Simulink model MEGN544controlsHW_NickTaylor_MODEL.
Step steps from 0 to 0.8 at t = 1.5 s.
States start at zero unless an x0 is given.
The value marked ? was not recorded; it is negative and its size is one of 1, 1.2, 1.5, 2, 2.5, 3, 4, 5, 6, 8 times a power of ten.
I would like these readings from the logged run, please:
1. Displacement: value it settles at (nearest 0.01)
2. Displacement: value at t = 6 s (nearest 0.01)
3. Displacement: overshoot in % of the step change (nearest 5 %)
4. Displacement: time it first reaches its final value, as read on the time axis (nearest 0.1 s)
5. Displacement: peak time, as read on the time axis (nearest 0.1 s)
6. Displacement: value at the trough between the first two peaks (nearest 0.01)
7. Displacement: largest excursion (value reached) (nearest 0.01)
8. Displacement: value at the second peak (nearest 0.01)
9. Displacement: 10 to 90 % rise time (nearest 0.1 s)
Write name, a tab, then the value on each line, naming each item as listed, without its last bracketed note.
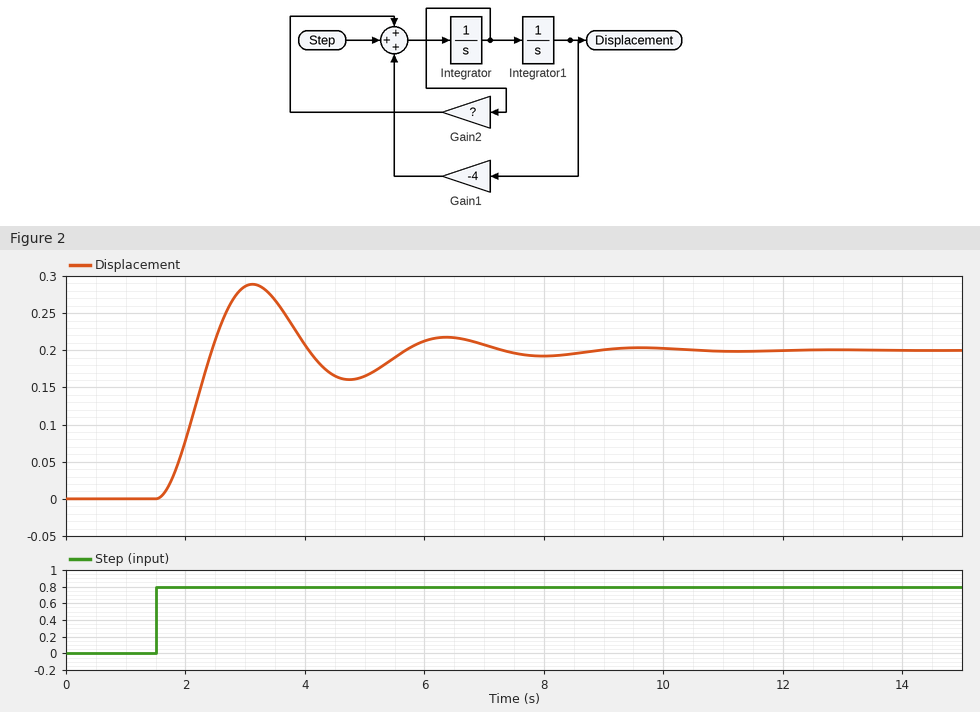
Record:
Displacement: value it settles at	0.20
Displacement: value at t = 6 s	0.21
Displacement: overshoot in % of the step change	45 %
Displacement: time it first reaches its final value, as read on the time axis	2.4 s
Displacement: peak time, as read on the time axis	3.1 s
Displacement: value at the trough between the first two peaks	0.16
Displacement: largest excursion (value reached)	0.29
Displacement: value at the second peak	0.22
Displacement: 10 to 90 % rise time	0.6 s
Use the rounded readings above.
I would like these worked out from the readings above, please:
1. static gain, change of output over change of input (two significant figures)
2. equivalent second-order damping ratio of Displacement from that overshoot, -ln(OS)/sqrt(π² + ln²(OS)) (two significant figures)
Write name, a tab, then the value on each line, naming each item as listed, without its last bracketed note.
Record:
static gain, change of output over change of input	0.25
equivalent second-order damping ratio of Displacement from that overshoot, -ln(OS)/sqrt(π² + ln²(OS))	0.25
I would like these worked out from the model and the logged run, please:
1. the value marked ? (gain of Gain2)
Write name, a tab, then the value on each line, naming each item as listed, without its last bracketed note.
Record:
the value marked ?	-1
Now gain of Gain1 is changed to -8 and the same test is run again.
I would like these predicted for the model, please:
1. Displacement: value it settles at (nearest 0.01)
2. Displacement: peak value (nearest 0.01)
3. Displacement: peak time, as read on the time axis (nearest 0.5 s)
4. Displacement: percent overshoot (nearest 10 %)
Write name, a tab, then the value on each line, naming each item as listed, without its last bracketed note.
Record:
Displacement: value it settles at	0.10
Displacement: peak value	0.16
Displacement: peak time, as read on the time axis	2.5 s
Displacement: percent overshoot	60 %
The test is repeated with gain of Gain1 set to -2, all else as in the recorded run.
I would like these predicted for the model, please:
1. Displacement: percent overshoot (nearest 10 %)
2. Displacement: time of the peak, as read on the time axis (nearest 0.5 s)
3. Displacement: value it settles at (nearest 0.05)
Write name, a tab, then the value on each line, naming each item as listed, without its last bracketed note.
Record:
Displacement: percent overshoot	30 %
Displacement: time of the peak, as read on the time axis	4.0 s
Displacement: value it settles at	0.40
